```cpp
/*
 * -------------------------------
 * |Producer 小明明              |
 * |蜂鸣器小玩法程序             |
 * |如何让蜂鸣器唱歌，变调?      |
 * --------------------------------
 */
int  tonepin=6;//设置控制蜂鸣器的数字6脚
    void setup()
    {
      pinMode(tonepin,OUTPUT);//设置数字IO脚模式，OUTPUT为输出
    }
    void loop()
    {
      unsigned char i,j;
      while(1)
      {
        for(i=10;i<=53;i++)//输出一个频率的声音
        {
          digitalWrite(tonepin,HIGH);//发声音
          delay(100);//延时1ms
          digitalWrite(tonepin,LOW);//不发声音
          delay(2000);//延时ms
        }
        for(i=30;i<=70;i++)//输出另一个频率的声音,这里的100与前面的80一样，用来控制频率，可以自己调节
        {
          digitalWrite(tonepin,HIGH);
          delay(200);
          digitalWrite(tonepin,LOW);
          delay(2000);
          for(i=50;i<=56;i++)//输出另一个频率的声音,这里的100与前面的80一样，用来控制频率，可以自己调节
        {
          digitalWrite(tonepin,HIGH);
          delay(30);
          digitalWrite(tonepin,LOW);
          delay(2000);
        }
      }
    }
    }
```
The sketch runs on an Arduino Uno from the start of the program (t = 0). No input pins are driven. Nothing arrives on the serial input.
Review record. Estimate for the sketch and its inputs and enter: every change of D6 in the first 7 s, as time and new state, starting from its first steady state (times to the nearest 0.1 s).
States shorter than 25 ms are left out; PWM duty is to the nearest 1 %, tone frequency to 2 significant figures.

0 s high; 0.1 s low; 2.1 s high; 2.2 s low; 4.2 s high; 4.3 s low; 6.3 s high; 6.4 s low
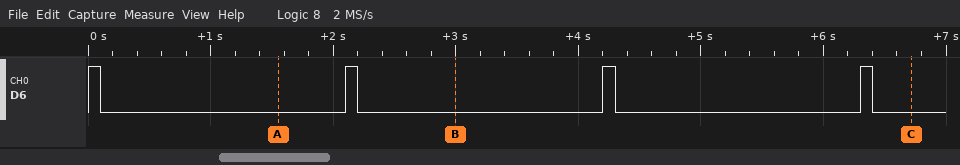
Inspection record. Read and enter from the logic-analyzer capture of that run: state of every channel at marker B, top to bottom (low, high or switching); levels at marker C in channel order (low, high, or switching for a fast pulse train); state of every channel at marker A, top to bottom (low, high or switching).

D6 low
D6 low
D6 low
